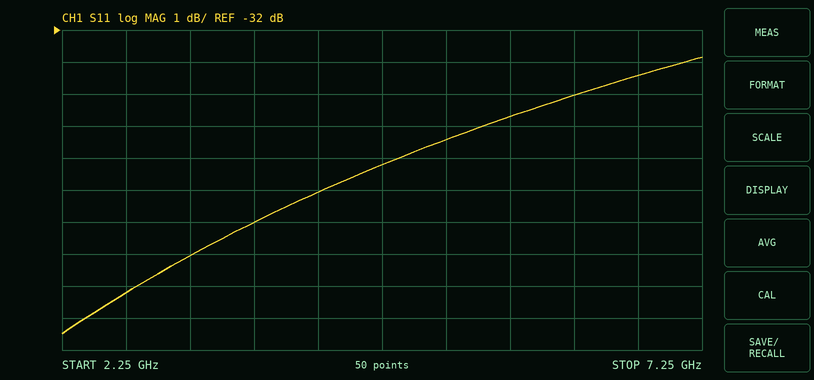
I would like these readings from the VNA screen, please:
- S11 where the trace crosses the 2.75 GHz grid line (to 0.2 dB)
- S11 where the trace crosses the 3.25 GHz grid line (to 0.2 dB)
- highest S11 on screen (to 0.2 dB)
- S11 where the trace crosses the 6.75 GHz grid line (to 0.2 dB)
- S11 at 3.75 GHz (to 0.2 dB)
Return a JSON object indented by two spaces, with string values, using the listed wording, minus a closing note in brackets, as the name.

{
  "S11 where the trace crosses the 2.75 GHz grid line": "-40.2 dB",
  "S11 where the trace crosses the 3.25 GHz grid line": "-39.0 dB",
  "highest S11 on screen": "-32.8 dB",
  "S11 where the trace crosses the 6.75 GHz grid line": "-33.4 dB",
  "S11 at 3.75 GHz": "-38.0 dB"
}
